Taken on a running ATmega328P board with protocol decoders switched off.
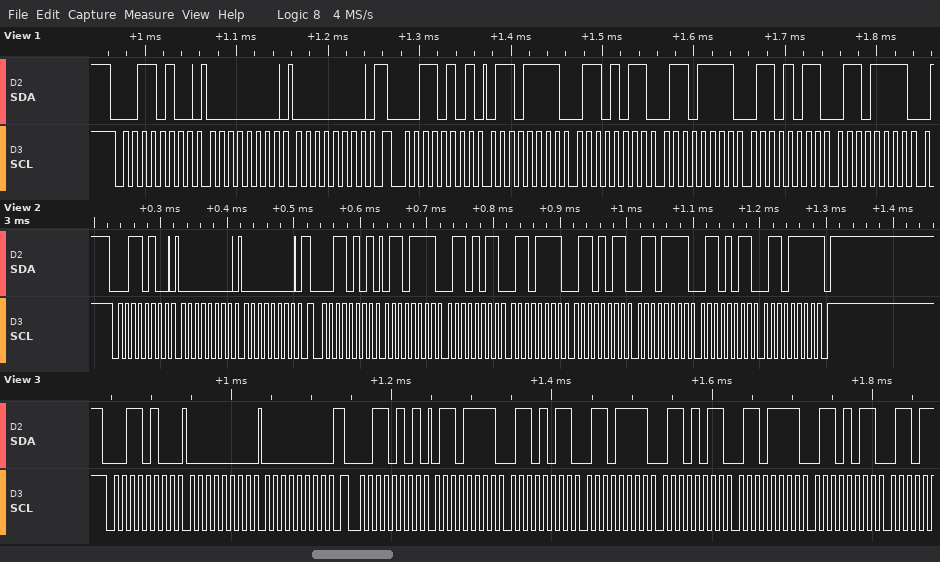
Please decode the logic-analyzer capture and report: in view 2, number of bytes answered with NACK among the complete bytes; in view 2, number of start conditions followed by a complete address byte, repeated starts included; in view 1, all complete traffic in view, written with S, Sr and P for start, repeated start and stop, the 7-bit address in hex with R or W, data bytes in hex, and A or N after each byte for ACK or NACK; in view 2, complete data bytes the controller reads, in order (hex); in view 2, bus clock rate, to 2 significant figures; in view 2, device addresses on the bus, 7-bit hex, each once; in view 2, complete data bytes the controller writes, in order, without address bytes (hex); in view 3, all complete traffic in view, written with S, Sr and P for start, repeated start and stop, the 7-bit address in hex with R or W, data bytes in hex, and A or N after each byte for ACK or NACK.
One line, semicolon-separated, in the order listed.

1; 2; S 1AW A 00 A 00 A Sr 1AR A 6F A 6B A 6F A 6B A 6F A; 6F 6B 6F 6B 6F 6B 6F; 100 kHz; 0x1A; 00 00; S 1AW A 00 A 00 A Sr 1AR A 6F A 6B A 6F A 6B A 6F A 6B A
